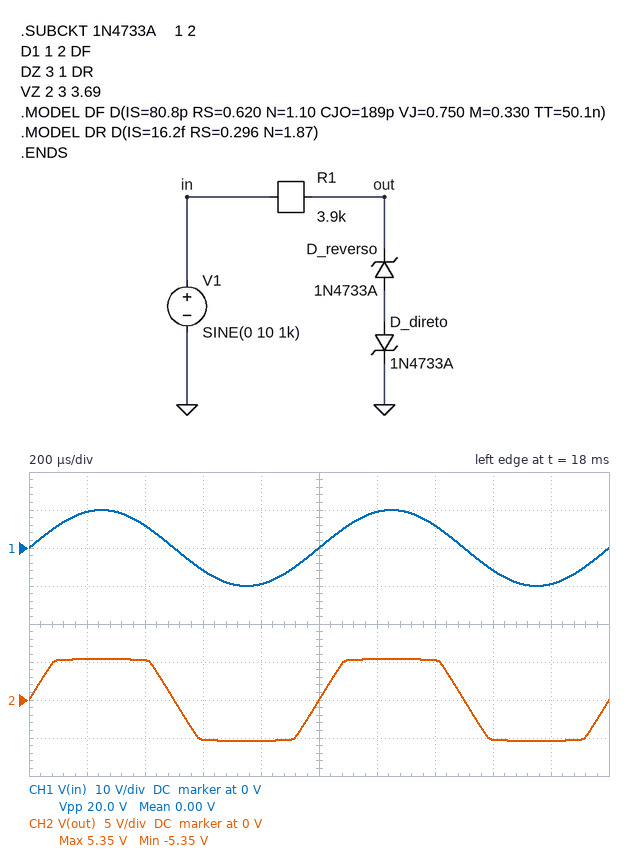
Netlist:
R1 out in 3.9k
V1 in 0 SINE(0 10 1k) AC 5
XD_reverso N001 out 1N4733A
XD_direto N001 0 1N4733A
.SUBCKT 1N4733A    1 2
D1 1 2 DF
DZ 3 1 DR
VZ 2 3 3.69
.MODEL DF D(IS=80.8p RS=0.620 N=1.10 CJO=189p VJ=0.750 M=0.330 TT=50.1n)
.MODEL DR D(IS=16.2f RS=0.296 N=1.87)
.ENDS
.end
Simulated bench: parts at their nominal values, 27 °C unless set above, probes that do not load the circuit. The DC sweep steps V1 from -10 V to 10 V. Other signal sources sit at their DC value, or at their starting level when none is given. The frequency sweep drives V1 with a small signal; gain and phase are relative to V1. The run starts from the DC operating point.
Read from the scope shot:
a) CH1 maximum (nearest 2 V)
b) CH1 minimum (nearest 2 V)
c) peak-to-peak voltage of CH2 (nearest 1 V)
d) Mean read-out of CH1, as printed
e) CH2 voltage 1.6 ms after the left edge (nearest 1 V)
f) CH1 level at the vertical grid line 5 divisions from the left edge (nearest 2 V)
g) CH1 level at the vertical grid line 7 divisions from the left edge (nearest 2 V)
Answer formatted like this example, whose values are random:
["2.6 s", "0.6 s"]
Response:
["10 V", "-10 V", "11 V", "0.00 V", "-5 V", "0 V", "6 V"]
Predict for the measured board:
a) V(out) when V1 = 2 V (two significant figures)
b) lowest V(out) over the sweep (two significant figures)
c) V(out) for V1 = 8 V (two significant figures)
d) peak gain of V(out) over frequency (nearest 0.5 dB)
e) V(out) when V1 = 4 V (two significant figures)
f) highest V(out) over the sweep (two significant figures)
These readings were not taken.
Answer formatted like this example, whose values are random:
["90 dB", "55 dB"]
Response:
["2.0 V", "-5.4 V", "5.3 V", "0 dB", "4.0 V", "5.4 V"]
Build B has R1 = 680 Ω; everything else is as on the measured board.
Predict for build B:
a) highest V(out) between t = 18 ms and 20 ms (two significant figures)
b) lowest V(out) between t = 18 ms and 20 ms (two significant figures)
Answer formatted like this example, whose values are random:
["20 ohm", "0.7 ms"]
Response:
["5.5 V", "-5.5 V"]
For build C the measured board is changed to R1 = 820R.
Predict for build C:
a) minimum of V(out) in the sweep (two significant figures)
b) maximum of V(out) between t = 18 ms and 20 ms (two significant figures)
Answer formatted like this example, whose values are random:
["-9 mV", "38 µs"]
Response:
["-5.5 V", "5.5 V"]
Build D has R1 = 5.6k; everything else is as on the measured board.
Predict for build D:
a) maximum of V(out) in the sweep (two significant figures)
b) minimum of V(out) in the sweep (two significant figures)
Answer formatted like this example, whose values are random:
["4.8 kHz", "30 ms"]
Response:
["5.3 V", "-5.3 V"]
